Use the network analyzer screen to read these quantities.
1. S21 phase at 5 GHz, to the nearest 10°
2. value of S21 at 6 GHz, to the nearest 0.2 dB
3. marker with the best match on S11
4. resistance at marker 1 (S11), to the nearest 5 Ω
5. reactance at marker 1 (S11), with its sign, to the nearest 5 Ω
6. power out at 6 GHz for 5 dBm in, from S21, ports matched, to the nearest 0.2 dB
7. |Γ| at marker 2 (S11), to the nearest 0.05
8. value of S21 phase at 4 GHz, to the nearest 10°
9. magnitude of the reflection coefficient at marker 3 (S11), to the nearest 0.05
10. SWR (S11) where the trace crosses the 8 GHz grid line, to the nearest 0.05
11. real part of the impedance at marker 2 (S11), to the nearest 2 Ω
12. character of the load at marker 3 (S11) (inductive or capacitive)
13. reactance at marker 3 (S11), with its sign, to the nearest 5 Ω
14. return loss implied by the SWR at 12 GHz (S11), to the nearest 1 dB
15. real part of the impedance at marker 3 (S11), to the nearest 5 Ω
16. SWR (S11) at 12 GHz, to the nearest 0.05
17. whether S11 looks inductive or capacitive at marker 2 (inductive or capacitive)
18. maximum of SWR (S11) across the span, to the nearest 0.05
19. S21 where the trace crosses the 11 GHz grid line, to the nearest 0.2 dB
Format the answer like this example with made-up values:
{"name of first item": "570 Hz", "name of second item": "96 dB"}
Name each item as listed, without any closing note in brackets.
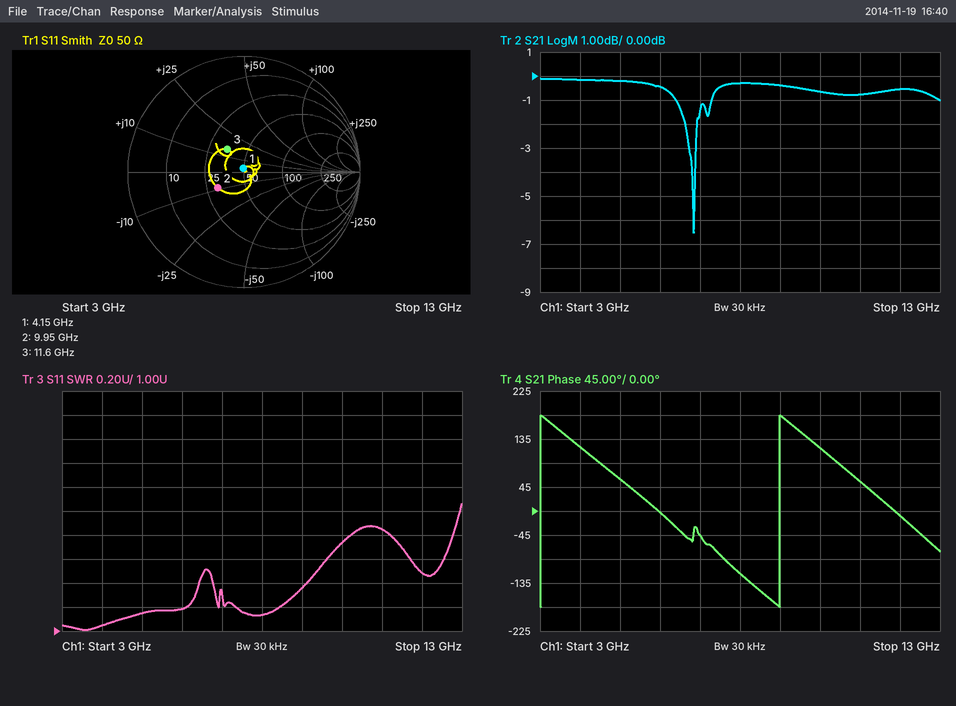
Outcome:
{"S21 phase at 5 GHz, to the nearest 10°": "60°", "value of S21 at 6 GHz, to the nearest 0.2 dB": "-0.4 dB", "marker with the best match on S11": "marker 1", "resistance at marker 1 (S11), to the nearest 5 Ω": "50 Ω", "reactance at marker 1 (S11), with its sign, to the nearest 5 Ω": "+5 Ω", "power out at 6 GHz for 5 dBm in, from S21, ports matched, to the nearest 0.2 dB": "4.6 dBm", "|Γ| at marker 2 (S11), to the nearest 0.05": "0.25", "value of S21 phase at 4 GHz, to the nearest 10°": "120°", "magnitude of the reflection coefficient at marker 3 (S11), to the nearest 0.05": "0.25", "SWR (S11) where the trace crosses the 8 GHz grid line, to the nearest 0.05": "1.15", "real part of the impedance at marker 2 (S11), to the nearest 2 Ω": "30 Ω", "character of the load at marker 3 (S11)": "inductive", "reactance at marker 3 (S11), with its sign, to the nearest 5 Ω": "+15 Ω", "return loss implied by the SWR at 12 GHz (S11), to the nearest 1 dB": "14 dB", "real part of the impedance at marker 3 (S11), to the nearest 5 Ω": "35 Ω", "SWR (S11) at 12 GHz, to the nearest 0.05": "1.50", "whether S11 looks inductive or capacitive at marker 2": "capacitive", "maximum of SWR (S11) across the span, to the nearest 0.05": "2.05", "S21 where the trace crosses the 11 GHz grid line, to the nearest 0.2 dB": "-0.8 dB"}
